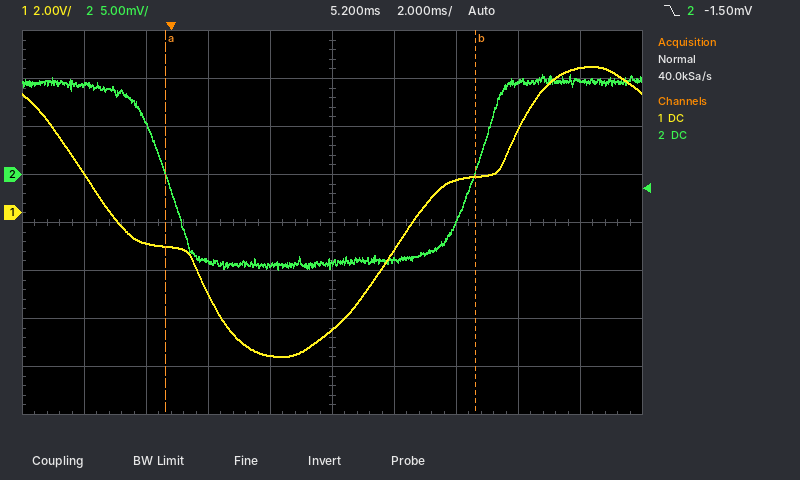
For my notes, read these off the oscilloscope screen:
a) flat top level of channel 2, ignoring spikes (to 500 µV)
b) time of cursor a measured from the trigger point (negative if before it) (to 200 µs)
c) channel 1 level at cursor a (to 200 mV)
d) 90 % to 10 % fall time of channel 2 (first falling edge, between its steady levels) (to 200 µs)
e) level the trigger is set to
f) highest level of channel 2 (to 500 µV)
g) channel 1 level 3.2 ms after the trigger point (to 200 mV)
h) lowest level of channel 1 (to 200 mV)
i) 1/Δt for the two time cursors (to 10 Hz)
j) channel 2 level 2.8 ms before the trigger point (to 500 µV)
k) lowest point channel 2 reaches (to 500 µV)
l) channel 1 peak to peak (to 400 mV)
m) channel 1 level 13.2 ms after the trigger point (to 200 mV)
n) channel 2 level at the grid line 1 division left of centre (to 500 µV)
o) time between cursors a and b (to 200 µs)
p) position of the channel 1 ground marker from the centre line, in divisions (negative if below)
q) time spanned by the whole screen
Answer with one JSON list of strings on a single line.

["9.5 mV", "-200 µs", "-1.4 V", "1.8 ms", "-1.50 mV", "10.5 mV", "-6.0 V", "-6.0 V", "100 Hz", "9.5 mV", "-10.0 mV", "12.0 V", "6.0 V", "-9.5 mV", "10.0 ms", "+0.2 div", "20 ms"]
